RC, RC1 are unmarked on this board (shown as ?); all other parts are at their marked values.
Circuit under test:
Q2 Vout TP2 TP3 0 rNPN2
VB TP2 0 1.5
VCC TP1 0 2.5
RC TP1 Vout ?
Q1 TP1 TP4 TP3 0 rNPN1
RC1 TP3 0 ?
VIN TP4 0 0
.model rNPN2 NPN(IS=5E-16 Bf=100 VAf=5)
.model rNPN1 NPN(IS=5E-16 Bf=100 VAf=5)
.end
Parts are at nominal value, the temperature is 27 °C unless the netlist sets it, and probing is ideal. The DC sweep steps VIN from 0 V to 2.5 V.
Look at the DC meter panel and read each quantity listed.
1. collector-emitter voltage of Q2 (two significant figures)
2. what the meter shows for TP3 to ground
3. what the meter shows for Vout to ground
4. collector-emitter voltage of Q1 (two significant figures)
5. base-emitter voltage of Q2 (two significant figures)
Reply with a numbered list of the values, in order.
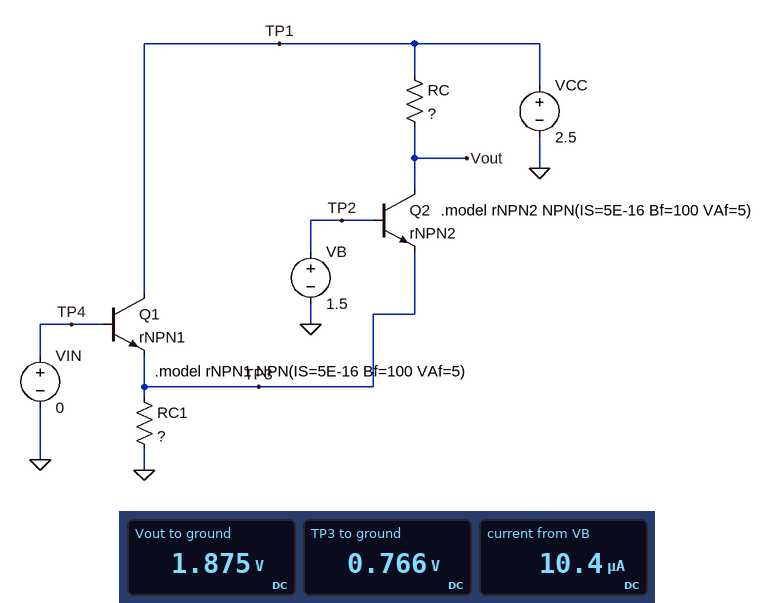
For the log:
1. 1.1 V
2. 0.766 V
3. 1.875 V
4. 1.7 V
5. 730 mV
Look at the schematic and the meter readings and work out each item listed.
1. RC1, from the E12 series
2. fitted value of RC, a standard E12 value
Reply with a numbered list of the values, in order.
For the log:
1. 680 Ω
2. 560 Ω
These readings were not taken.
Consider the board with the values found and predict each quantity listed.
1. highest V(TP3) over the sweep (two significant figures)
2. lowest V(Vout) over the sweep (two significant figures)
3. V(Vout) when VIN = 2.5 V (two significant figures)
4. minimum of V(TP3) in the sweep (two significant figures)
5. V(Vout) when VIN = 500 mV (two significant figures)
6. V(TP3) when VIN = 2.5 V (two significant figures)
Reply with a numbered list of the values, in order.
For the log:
1. 1.7 V
2. 1.9 V
3. 2.5 V
4. 770 mV
5. 1.9 V
6. 1.7 V
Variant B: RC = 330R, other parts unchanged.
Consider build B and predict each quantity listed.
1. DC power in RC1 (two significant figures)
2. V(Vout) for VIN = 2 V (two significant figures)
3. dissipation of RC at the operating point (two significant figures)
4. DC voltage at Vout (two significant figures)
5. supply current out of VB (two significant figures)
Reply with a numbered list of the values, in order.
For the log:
1. 870 µW
2. 2.5 V
3. 410 µW
4. 2.1 V
5. 9.9 µA
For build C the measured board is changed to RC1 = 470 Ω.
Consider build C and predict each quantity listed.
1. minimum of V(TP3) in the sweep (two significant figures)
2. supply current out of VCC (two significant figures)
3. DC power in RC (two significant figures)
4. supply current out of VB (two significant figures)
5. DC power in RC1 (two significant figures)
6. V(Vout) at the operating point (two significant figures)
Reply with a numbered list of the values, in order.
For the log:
1. 760 mV
2. 1.6 mA
3. 1.4 mW
4. 16 µA
5. 1.2 mW
6. 1.6 V
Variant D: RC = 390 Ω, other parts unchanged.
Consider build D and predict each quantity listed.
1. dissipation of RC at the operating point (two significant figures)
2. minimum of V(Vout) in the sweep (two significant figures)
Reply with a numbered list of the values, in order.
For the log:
1. 490 µW
2. 2.1 V
